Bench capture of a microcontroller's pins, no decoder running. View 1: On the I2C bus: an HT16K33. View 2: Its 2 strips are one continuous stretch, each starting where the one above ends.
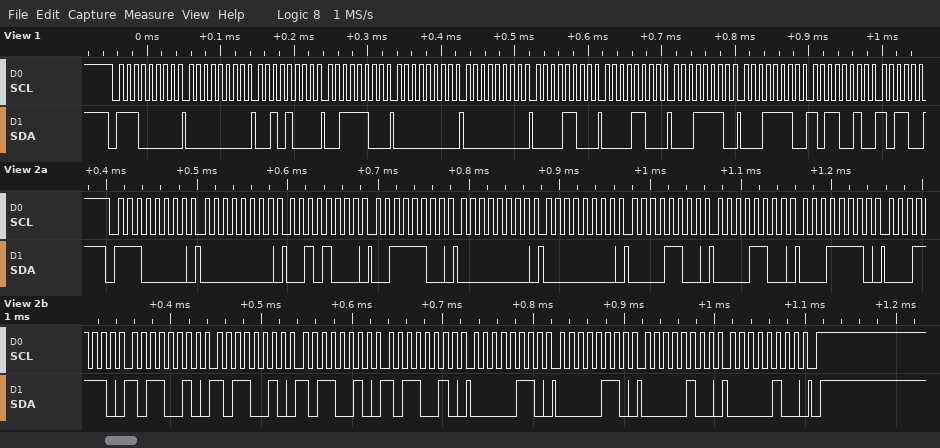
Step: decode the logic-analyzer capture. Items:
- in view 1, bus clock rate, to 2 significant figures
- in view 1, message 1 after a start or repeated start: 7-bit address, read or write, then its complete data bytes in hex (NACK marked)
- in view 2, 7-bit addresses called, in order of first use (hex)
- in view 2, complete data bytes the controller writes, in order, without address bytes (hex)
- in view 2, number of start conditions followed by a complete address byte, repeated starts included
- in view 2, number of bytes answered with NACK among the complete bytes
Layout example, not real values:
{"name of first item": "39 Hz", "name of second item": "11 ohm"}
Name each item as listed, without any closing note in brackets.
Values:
{"in view 1, bus clock rate, to 2 significant figures": "100 kHz", "in view 1, message 1 after a start or repeated start: 7-bit address, read or write, then its complete data bytes in hex": "0x70 write: 00 28 3C 00 00 0C 0C 1E 1E B2", "in view 2, 7-bit addresses called, in order of first use": "0x70", "in view 2, complete data bytes the controller writes, in order, without address bytes": "00 28 3C 00 00 0C 0C 1E 1E B2 B2 B2 B2 06 06 04 04", "in view 2, number of start conditions followed by a complete address byte, repeated starts included": "1", "in view 2, number of bytes answered with NACK among the complete bytes": "0"}
